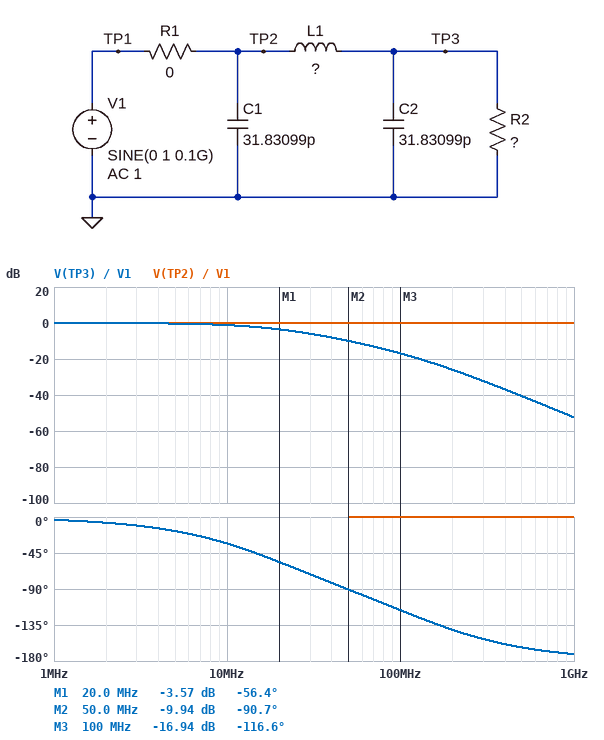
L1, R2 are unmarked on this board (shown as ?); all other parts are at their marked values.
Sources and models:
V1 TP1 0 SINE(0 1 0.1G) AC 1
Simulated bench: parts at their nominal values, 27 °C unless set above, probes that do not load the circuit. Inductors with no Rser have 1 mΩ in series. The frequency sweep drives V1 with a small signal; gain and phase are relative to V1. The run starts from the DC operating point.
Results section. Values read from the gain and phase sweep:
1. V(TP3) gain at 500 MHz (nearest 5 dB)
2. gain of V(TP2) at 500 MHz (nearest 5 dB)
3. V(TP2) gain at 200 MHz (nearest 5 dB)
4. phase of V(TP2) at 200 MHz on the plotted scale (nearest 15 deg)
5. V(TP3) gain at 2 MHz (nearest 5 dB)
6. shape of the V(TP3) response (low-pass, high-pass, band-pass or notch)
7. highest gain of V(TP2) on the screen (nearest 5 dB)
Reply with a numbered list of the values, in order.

1. -40 dB
2. 0 dB
3. 0 dB
4. 0 deg
5. 0 dB
6. low-pass
7. 0 dB
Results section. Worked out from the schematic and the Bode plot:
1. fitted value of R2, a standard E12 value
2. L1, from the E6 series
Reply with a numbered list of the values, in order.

1. 33 Ω
2. 330 nH
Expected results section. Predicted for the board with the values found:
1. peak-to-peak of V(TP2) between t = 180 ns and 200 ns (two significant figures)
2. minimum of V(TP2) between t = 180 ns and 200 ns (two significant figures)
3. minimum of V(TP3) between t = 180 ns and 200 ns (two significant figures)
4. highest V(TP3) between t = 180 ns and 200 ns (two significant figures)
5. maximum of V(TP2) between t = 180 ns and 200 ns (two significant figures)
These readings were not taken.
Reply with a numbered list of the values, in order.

1. 2.0 V
2. -1.0 V
3. -140 mV
4. 140 mV
5. 1.0 V
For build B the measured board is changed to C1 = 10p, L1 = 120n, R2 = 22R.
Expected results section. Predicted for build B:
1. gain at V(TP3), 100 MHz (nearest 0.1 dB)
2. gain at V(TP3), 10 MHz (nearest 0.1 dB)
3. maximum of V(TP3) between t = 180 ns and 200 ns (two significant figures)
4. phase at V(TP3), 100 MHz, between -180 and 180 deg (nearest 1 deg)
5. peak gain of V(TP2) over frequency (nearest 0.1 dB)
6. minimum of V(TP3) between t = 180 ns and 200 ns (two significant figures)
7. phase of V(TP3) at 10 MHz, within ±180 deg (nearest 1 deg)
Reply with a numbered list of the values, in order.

1. -10.8 dB
2. -0.4 dB
3. 290 mV
4. -98 deg
5. 0 dB
6. -290 mV
7. -19 deg
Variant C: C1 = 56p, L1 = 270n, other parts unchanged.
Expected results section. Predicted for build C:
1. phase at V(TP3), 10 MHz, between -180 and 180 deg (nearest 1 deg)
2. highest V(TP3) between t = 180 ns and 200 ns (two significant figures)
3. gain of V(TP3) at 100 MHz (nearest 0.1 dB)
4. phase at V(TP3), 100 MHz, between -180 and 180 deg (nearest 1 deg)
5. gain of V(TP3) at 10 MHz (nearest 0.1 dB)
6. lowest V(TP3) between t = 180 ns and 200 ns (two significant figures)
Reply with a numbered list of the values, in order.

1. -28 deg
2. 180 mV
3. -15.1 dB
4. -115 deg
5. -0.8 dB
6. -180 mV
